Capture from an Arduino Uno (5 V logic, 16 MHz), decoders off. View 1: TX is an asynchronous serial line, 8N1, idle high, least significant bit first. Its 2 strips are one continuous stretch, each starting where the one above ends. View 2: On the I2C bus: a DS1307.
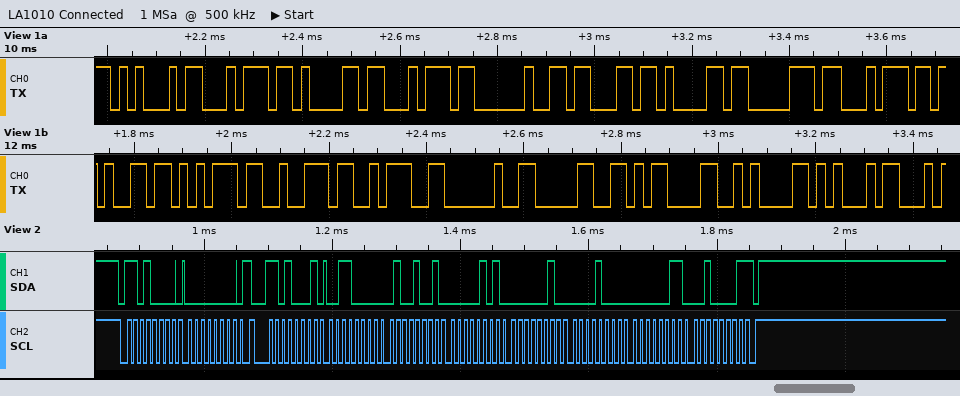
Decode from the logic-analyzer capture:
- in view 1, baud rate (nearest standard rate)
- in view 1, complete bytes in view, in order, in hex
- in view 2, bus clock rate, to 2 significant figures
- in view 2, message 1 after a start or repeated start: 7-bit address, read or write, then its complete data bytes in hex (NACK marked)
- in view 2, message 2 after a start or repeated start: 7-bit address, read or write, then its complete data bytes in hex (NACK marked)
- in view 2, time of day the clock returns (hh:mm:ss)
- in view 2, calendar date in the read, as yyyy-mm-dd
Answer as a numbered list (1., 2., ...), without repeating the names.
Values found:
1. 57600 baud
2. 45 74 61 74 20 63 61 70 74 65 75 72 3A 20 30 0D 0A 45
3. 100 kHz
4. 0x68 write: 00
5. 0x68 read: 30 49 05 02 08 03 21 NACK
6. 05:49:30
7. 2021-03-08
